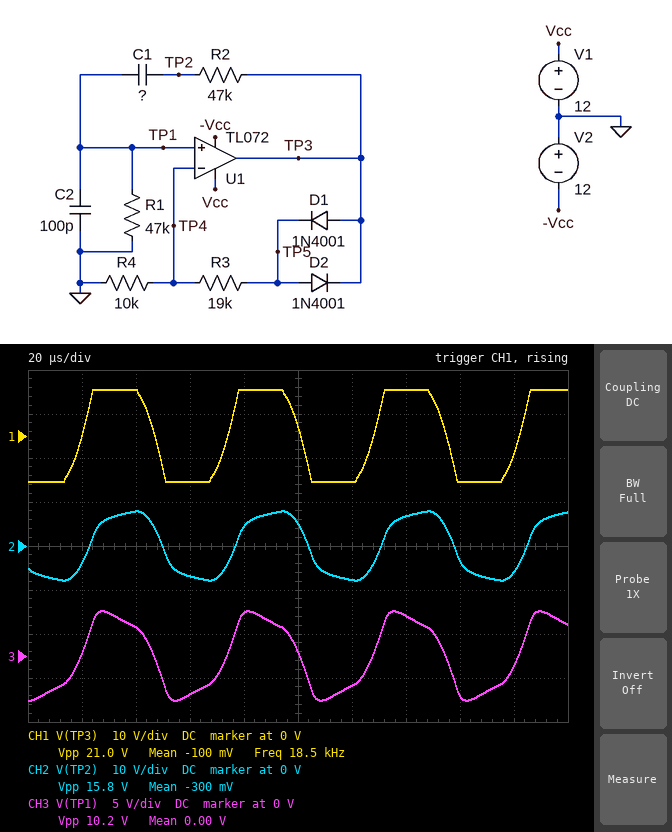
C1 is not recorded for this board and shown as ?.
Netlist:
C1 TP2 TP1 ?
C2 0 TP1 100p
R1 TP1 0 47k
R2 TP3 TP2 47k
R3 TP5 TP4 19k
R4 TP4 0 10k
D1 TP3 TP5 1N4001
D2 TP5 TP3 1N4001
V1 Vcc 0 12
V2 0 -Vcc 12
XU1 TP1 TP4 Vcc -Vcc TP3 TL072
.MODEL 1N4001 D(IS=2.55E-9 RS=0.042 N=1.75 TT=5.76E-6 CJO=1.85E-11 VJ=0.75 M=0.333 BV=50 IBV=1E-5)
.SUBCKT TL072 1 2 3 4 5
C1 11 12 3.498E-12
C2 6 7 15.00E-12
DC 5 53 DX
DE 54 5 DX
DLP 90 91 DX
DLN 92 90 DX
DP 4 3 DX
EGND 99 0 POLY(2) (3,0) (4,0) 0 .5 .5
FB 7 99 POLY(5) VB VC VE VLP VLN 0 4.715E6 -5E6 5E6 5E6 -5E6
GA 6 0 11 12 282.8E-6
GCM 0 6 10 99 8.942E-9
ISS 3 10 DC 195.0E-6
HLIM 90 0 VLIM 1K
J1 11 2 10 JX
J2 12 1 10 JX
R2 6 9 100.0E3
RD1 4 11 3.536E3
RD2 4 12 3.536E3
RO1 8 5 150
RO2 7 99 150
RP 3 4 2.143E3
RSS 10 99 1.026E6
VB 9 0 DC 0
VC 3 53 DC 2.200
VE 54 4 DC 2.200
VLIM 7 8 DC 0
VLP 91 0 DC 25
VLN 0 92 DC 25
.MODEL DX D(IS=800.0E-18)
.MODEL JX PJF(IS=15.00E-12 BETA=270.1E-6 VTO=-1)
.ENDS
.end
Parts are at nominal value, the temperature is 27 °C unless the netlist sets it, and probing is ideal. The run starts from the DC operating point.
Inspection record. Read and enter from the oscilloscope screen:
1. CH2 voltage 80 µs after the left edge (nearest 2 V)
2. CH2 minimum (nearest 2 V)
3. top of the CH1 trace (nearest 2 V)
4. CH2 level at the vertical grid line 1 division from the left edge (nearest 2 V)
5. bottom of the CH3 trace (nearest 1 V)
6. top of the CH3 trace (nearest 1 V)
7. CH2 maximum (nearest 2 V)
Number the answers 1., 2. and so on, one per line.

1. 4 V
2. -8 V
3. 10 V
4. -4 V
5. -5 V
6. 5 V
7. 8 V
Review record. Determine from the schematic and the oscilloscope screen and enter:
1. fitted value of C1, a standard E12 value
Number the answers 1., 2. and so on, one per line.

1. 220 pF
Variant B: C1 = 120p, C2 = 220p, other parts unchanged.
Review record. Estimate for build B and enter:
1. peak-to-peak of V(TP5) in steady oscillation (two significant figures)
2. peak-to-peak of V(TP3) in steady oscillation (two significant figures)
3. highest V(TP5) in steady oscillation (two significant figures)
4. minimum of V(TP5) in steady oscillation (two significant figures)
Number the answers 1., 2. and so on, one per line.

1. 2.9 V
2. 3.8 V
3. 1.5 V
4. -1.5 V
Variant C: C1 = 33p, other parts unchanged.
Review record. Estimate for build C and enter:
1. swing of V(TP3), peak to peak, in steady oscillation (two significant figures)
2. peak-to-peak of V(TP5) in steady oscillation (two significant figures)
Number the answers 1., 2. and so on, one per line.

1. 1.5 V
2. 790 mV
